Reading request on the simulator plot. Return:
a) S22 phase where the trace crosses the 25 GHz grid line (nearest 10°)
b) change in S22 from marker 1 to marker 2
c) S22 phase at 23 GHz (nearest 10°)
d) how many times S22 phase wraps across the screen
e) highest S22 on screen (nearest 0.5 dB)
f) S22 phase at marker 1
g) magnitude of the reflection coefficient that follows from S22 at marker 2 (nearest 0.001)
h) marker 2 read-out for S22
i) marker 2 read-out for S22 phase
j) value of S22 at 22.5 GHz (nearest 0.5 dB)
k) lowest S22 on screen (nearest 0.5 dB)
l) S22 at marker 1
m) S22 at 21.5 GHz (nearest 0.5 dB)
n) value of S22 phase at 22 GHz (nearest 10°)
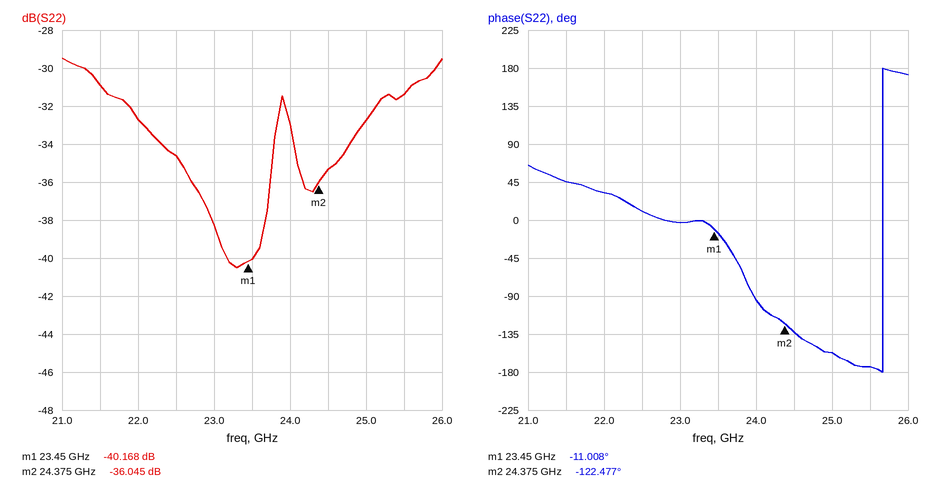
-160°
4.123 dB
0°
1
-29.5 dB
-11.008°
0.016
-36.045 dB
-122.477°
-34.5 dB
-40.5 dB
-40.168 dB
-31.0 dB
30°
